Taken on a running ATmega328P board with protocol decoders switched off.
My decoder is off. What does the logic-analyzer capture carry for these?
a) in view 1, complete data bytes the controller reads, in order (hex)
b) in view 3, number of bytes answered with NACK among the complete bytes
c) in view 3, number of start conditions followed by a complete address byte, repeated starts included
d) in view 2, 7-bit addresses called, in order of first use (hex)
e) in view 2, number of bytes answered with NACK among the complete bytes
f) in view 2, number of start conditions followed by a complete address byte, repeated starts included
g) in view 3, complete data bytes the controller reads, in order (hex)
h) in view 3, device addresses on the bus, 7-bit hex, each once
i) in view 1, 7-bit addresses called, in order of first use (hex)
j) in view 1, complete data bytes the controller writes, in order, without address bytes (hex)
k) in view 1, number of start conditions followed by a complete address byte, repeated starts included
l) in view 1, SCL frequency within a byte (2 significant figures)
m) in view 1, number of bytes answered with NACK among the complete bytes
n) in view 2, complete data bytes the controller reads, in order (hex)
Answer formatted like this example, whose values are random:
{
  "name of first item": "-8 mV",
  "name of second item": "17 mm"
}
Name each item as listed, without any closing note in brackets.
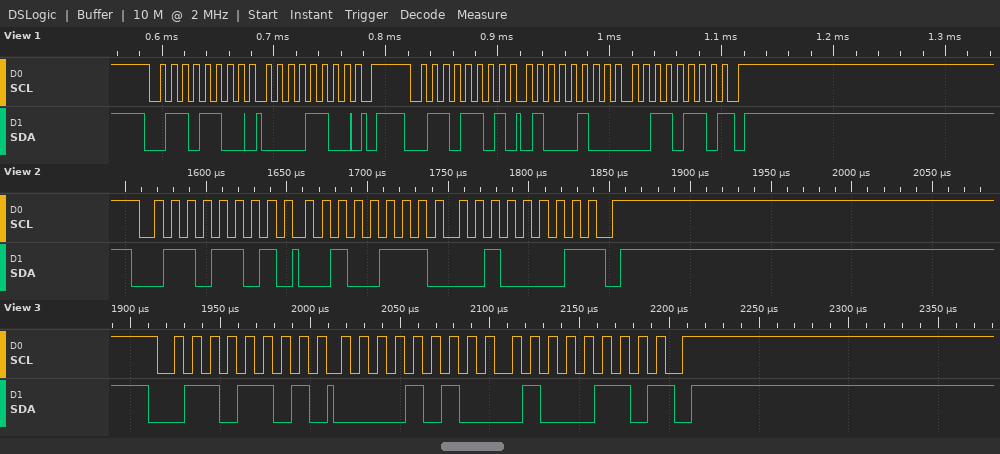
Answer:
{
  "in view 1, complete data bytes the controller reads, in order": "44 36",
  "in view 3, number of bytes answered with NACK among the complete bytes": "1",
  "in view 3, number of start conditions followed by a complete address byte, repeated starts included": "1",
  "in view 2, 7-bit addresses called, in order of first use": "0x36",
  "in view 2, number of bytes answered with NACK among the complete bytes": "1",
  "in view 2, number of start conditions followed by a complete address byte, repeated starts included": "1",
  "in view 3, complete data bytes the controller reads, in order": "0A 46",
  "in view 3, device addresses on the bus, 7-bit hex, each once": "0x36",
  "in view 1, 7-bit addresses called, in order of first use": "0x36",
  "in view 1, complete data bytes the controller writes, in order, without address bytes": "0C",
  "in view 1, number of start conditions followed by a complete address byte, repeated starts included": "2",
  "in view 1, SCL frequency within a byte": "100 kHz",
  "in view 1, number of bytes answered with NACK among the complete bytes": "1",
  "in view 2, complete data bytes the controller reads, in order": "27 21"
}
